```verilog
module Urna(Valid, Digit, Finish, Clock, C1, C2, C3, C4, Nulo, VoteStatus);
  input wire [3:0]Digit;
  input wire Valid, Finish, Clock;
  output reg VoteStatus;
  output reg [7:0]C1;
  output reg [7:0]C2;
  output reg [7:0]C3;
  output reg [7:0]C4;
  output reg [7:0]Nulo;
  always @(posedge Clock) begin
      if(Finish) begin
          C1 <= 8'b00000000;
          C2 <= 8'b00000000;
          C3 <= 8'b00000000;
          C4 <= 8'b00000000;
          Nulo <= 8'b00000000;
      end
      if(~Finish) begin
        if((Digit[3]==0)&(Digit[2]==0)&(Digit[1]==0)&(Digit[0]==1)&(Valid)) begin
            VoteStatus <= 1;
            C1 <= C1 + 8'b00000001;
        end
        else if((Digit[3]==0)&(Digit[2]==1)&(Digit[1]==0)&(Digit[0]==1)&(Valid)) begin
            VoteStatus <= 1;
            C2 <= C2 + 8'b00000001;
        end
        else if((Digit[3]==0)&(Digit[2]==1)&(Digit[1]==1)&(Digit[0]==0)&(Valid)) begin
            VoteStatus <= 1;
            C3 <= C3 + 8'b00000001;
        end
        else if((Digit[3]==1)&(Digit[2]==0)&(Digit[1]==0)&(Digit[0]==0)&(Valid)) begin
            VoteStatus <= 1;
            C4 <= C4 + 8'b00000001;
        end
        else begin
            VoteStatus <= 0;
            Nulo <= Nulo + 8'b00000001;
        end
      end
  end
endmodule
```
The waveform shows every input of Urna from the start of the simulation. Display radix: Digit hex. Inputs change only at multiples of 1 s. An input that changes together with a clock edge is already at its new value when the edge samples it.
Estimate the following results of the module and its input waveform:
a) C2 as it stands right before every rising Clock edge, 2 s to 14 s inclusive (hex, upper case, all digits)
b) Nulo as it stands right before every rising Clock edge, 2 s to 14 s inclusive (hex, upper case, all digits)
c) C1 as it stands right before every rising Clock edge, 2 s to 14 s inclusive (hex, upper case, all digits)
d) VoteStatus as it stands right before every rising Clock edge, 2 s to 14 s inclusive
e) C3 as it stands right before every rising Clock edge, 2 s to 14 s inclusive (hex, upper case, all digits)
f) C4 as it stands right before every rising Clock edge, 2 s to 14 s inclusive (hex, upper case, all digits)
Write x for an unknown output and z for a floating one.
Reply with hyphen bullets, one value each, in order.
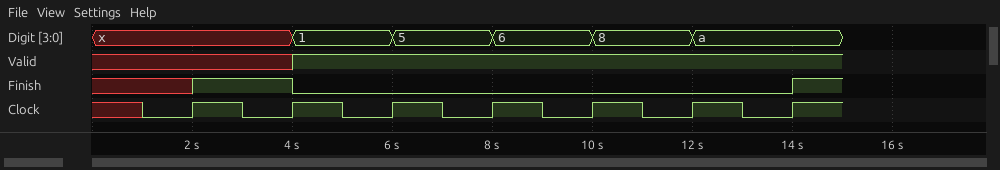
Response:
- x, 00, 00, 01, 01, 01, 01
- x, 00, 00, 00, 00, 00, 01
- x, 00, 01, 01, 01, 01, 01
- x x 1 1 1 1 0
- x, 00, 00, 00, 01, 01, 01
- x, 00, 00, 00, 00, 01, 01
